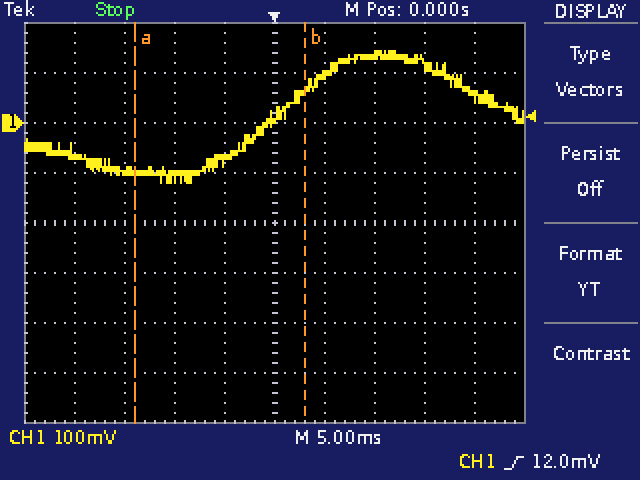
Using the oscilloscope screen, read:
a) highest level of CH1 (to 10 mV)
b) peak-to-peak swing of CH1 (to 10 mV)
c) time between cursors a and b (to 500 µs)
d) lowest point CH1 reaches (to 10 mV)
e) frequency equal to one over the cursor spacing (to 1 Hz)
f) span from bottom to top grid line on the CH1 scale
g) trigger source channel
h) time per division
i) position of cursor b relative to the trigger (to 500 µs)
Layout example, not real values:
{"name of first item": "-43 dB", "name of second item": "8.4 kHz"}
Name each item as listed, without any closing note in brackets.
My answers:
{"highest level of CH1": "140 mV", "peak-to-peak swing of CH1": "260 mV", "time between cursors a and b": "17.0 ms", "lowest point CH1 reaches": "-120 mV", "frequency equal to one over the cursor spacing": "59 Hz", "span from bottom to top grid line on the CH1 scale": "800 mV", "trigger source channel": "CH1", "time per division": "5 ms", "position of cursor b relative to the trigger": "+3.0 ms"}
